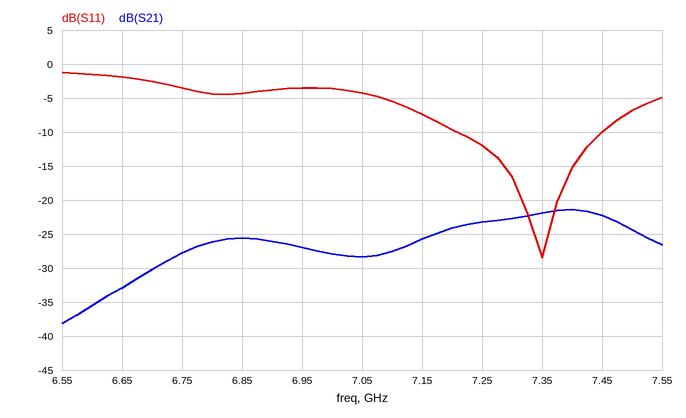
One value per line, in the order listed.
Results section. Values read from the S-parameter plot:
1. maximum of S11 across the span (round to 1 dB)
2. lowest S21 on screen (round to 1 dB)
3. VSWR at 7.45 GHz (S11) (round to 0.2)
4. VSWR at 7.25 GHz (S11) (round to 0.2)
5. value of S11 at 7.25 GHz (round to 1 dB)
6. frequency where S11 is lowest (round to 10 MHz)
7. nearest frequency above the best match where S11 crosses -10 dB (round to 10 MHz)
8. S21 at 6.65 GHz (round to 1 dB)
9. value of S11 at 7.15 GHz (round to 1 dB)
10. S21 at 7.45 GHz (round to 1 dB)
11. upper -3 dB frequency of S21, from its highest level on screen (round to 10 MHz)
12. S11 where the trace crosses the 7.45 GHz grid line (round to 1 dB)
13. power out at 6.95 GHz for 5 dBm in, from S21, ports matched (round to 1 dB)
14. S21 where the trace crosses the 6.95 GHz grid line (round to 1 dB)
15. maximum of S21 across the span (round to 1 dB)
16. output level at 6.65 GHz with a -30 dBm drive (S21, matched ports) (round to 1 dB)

-1 dB
-38 dB
2.0
1.6
-12 dB
7.35 GHz
7.45 GHz
-33 dB
-7 dB
-22 dB
7.50 GHz
-10 dB
-22 dBm
-27 dB
-21 dB
-63 dBm
